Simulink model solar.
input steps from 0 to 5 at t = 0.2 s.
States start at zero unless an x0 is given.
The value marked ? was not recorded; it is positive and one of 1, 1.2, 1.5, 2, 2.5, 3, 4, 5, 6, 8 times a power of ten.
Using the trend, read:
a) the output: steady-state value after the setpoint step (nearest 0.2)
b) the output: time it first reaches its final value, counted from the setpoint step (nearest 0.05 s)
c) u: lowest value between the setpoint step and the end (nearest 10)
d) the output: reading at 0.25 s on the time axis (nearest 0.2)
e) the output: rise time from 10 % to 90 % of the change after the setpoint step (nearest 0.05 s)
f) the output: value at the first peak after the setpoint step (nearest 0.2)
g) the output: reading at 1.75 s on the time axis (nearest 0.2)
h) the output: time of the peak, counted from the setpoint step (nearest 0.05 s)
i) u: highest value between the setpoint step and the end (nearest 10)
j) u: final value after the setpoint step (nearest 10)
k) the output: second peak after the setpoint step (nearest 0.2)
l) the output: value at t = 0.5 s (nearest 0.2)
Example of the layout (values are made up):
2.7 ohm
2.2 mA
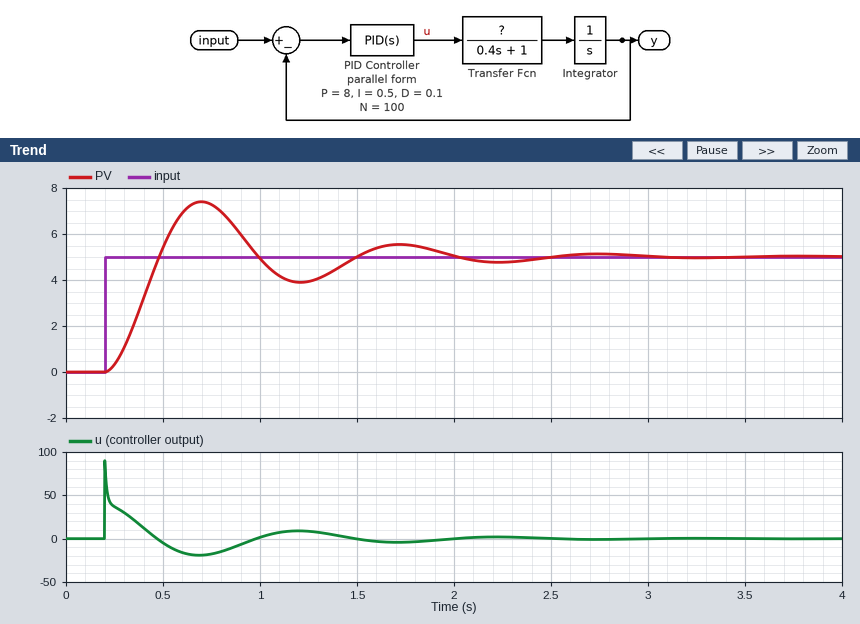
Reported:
5.0
0.30 s
-20
0.4
0.20 s
7.4
5.6
0.50 s
90
0
5.6
5.4
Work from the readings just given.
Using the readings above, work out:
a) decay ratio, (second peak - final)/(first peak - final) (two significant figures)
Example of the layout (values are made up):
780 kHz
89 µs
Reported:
0.25
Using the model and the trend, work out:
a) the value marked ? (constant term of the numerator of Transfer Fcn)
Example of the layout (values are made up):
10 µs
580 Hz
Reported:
2
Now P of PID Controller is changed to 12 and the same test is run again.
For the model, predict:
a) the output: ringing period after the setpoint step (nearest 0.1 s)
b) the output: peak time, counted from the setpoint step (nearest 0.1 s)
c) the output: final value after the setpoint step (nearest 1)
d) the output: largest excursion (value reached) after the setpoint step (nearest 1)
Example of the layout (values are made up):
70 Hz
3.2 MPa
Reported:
0.8 s
0.4 s
5
8
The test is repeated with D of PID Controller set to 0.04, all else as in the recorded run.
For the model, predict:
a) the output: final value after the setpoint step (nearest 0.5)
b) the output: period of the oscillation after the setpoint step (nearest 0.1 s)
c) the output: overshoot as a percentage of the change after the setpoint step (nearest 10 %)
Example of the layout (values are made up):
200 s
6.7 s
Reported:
5.0
1.0 s
50 %
